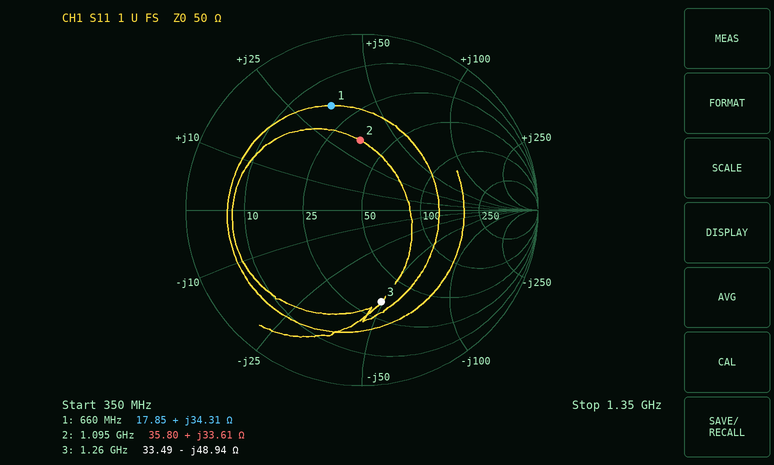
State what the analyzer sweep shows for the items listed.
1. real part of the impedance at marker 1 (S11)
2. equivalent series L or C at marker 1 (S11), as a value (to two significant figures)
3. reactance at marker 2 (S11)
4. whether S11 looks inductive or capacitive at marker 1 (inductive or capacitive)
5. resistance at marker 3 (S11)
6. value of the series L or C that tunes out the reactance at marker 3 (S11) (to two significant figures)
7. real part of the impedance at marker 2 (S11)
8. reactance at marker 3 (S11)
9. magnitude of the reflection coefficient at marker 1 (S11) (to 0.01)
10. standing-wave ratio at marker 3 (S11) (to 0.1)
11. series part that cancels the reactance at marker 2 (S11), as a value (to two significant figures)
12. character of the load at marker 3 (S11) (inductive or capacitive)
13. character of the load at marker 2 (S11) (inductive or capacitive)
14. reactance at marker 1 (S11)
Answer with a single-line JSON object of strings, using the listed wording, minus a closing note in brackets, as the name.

{"real part of the impedance at marker 1": "17.85 Ω", "equivalent series L or C at marker 1 (S11), as a value": "8.3 nH", "reactance at marker 2": "+33.61 Ω", "whether S11 looks inductive or capacitive at marker 1": "inductive", "resistance at marker 3": "33.49 Ω", "value of the series L or C that tunes out the reactance at marker 3 (S11)": "6.2 nH", "real part of the impedance at marker 2": "35.80 Ω", "reactance at marker 3": "-48.94 Ω", "magnitude of the reflection coefficient at marker 1 (S11)": "0.62", "standing-wave ratio at marker 3 (S11)": "3.3", "series part that cancels the reactance at marker 2 (S11), as a value": "4.3 pF", "character of the load at marker 3 (S11)": "capacitive", "character of the load at marker 2 (S11)": "inductive", "reactance at marker 1": "+34.31 Ω"}
